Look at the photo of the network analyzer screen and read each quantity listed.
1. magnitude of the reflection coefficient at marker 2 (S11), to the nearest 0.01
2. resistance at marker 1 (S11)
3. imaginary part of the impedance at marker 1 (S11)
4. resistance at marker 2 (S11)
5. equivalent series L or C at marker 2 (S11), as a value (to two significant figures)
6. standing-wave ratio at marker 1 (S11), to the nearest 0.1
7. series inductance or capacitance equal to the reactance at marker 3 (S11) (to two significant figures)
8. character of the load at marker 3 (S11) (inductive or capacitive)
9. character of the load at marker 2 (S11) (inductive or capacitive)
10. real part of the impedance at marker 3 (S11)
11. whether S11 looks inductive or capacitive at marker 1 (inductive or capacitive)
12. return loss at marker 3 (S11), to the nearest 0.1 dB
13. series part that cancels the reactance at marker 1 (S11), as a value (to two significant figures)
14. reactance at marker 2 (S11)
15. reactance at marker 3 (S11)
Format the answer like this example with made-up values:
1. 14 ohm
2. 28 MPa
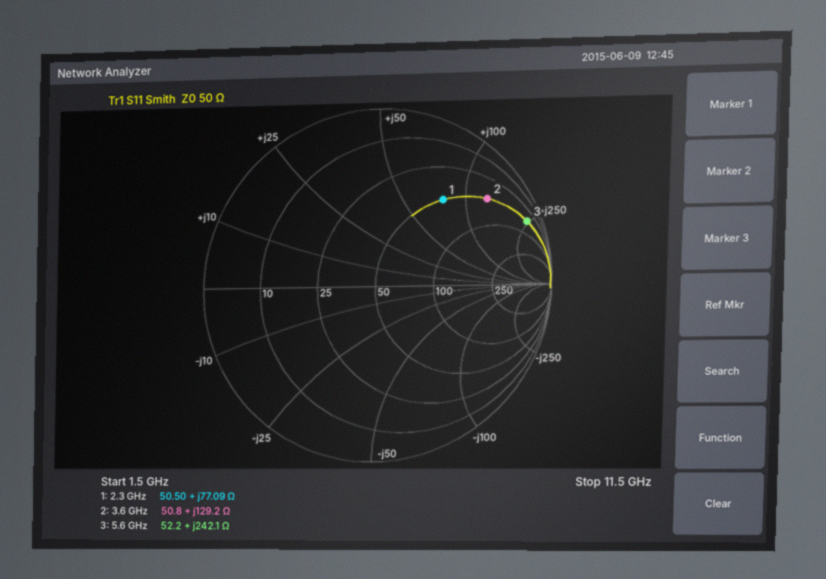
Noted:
1. 0.79
2. 50.50 Ω
3. +77.09 Ω
4. 50.8 Ω
5. 5.7 nH
6. 4.1
7. 6.9 nH
8. inductive
9. inductive
10. 52.2 Ω
11. inductive
12. 0.7 dB
13. 900 fF
14. +129.2 Ω
15. +242.1 Ω
